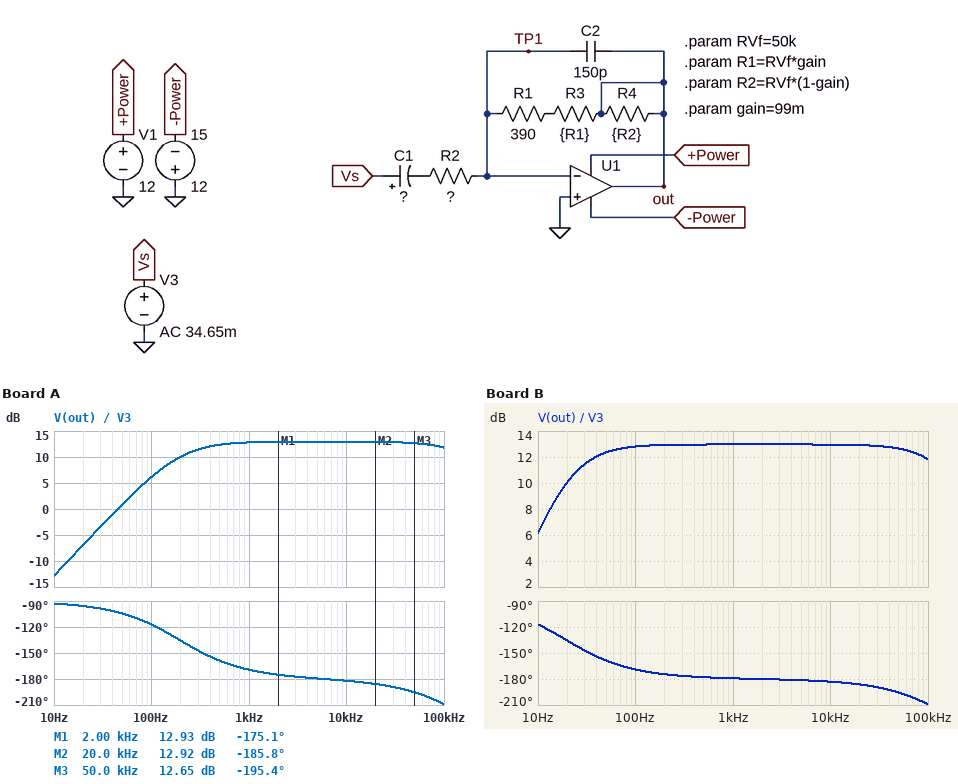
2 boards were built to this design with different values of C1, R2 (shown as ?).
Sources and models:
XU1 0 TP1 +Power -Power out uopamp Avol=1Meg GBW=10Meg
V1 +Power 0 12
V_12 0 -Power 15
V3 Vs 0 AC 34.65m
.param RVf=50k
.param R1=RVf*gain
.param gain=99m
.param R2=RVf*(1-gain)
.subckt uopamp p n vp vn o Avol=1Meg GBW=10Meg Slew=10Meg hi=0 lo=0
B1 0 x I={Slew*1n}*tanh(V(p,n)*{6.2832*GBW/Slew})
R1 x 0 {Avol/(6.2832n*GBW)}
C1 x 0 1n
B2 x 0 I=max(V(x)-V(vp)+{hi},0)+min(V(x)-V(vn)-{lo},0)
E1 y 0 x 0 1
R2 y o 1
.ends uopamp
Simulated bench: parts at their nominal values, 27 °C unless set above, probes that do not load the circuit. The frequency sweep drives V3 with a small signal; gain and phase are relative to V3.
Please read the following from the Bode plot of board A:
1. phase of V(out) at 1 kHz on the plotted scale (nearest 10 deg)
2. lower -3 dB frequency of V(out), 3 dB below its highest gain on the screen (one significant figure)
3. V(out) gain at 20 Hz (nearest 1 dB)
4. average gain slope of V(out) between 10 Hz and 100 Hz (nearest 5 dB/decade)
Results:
-170 deg
200 Hz
-7 dB
20 dB/decade
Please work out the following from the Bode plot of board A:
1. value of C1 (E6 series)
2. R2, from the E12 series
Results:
680 nF
1.2 kΩ
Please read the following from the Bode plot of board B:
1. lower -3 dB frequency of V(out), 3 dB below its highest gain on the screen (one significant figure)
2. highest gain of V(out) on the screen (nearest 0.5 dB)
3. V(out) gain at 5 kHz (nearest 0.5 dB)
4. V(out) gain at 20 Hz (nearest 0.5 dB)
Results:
20 Hz
13.0 dB
13.0 dB
10.0 dB
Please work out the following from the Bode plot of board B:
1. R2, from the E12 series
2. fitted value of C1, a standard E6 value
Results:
1.2 kΩ
6.8 µF
